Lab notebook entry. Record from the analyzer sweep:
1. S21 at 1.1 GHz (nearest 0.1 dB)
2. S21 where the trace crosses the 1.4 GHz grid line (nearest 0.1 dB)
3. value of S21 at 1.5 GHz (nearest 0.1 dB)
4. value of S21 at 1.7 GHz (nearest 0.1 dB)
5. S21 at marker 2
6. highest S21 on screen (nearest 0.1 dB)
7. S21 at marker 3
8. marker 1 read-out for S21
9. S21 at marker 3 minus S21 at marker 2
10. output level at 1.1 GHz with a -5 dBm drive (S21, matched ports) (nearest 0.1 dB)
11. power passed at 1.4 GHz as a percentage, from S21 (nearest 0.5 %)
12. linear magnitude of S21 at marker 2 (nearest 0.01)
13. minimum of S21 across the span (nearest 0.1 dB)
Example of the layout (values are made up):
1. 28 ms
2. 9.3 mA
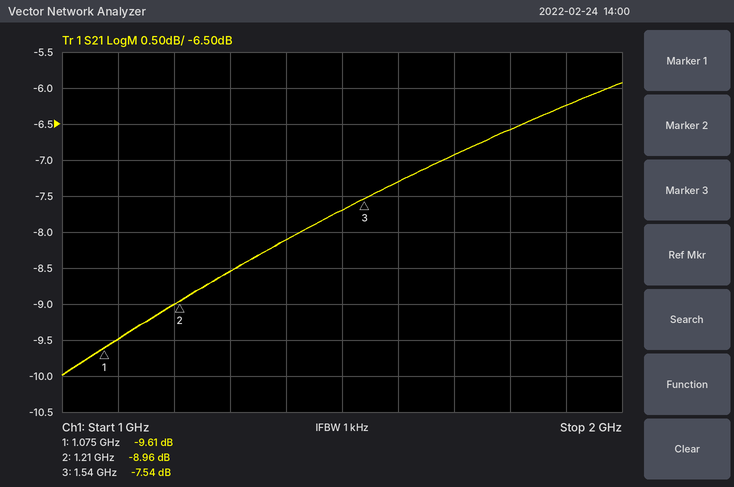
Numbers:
1. -9.5 dB
2. -8.1 dB
3. -7.7 dB
4. -6.9 dB
5. -8.96 dB
6. -5.9 dB
7. -7.54 dB
8. -9.61 dB
9. 1.42 dB
10. -14.5 dBm
11. 15.5 %
12. 0.36
13. -10.0 dB
